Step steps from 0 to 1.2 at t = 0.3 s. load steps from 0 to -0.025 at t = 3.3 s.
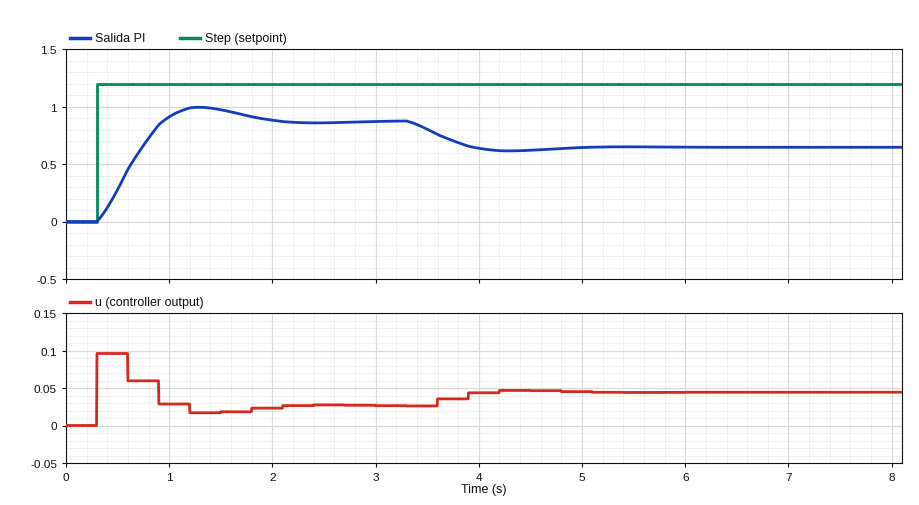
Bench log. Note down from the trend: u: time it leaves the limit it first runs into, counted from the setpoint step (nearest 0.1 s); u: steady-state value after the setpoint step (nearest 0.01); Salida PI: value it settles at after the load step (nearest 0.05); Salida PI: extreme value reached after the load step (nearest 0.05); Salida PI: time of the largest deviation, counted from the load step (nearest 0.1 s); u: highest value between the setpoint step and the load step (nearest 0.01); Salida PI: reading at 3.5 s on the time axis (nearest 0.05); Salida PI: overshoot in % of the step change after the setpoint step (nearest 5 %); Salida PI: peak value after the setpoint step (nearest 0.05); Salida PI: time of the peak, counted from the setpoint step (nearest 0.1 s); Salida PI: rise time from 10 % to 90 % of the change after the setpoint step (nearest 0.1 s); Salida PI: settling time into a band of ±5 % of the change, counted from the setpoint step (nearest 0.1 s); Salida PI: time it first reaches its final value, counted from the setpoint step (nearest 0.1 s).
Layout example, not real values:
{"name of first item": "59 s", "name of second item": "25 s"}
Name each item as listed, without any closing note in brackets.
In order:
{"u: time it leaves the limit it first runs into, counted from the setpoint step": "0.3 s", "u: steady-state value after the setpoint step": "0.03", "Salida PI: value it settles at after the load step": "0.65", "Salida PI: extreme value reached after the load step": "0.60", "Salida PI: time of the largest deviation, counted from the load step": "1.0 s", "u: highest value between the setpoint step and the load step": "0.10", "Salida PI: reading at 3.5 s on the time axis": "0.80", "Salida PI: overshoot in % of the step change after the setpoint step": "15 %", "Salida PI: peak value after the setpoint step": "1.00", "Salida PI: time of the peak, counted from the setpoint step": "1.0 s", "Salida PI: rise time from 10 % to 90 % of the change after the setpoint step": "0.5 s", "Salida PI: settling time into a band of ±5 % of the change, counted from the setpoint step": "1.5 s", "Salida PI: time it first reaches its final value, counted from the setpoint step": "0.6 s"}
